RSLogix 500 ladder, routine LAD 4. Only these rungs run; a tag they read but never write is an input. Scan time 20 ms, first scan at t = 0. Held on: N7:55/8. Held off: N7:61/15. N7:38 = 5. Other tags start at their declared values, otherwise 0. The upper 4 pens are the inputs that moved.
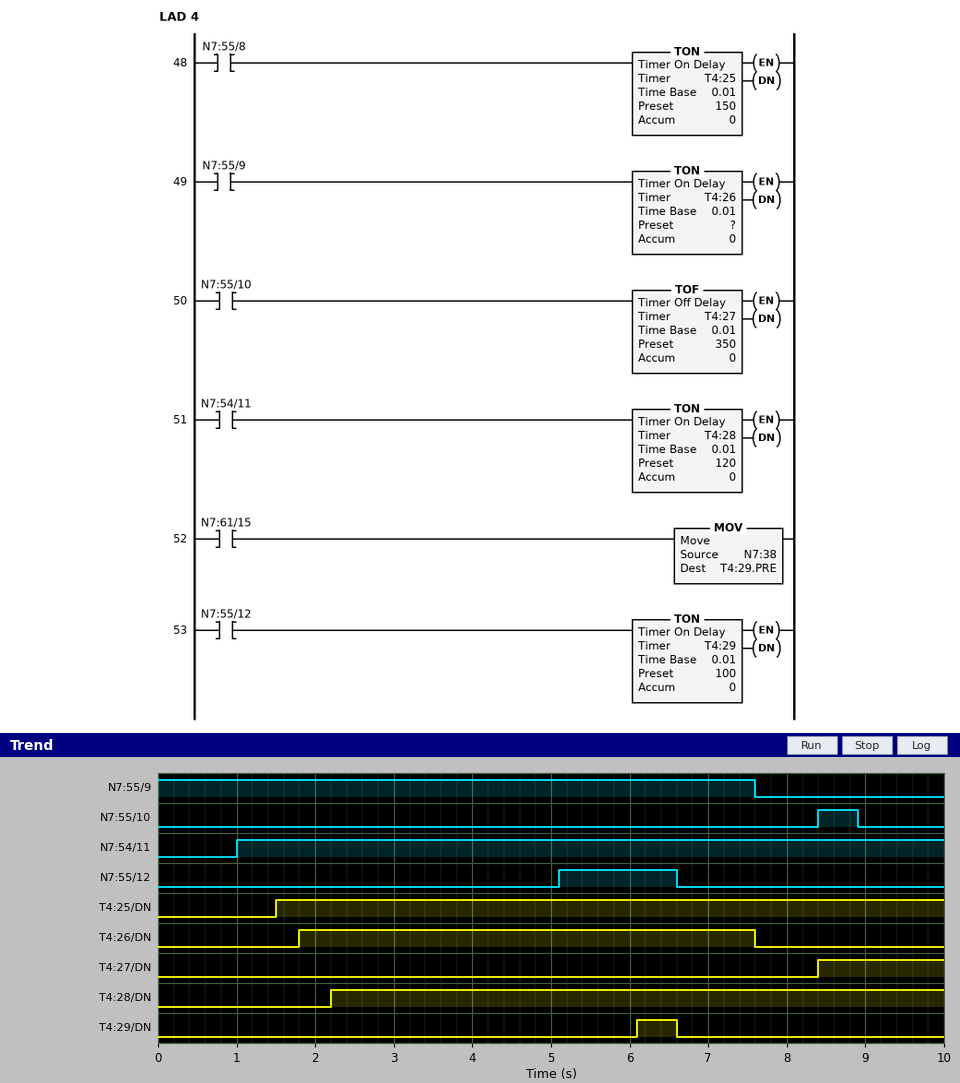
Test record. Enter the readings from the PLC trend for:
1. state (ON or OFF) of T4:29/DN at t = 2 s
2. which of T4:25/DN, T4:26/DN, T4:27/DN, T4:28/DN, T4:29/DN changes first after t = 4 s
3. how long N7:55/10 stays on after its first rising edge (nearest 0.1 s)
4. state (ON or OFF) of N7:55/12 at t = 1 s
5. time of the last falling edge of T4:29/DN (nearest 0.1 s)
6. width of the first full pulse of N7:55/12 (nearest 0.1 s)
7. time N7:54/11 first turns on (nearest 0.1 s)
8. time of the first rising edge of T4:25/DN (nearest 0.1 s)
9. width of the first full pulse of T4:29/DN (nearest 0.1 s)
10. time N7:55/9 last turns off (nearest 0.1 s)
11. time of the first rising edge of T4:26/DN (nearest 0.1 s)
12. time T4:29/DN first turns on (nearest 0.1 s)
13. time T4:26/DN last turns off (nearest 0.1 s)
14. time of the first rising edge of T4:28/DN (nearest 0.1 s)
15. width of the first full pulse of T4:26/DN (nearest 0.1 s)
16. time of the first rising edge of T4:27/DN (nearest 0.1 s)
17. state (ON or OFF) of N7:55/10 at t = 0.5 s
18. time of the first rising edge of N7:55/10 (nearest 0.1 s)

OFF
T4:29/DN
0.5 s
OFF
6.6 s
1.5 s
1.0 s
1.5 s
0.5 s
7.6 s
1.8 s
6.1 s
7.6 s
2.2 s
5.8 s
8.4 s
OFF
8.4 s
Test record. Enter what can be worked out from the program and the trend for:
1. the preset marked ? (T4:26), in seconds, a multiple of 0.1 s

1.8 s
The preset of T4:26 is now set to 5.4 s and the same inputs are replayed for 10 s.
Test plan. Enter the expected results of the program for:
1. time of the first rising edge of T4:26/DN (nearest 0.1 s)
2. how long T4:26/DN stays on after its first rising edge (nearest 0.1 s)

5.4 s
2.2 s
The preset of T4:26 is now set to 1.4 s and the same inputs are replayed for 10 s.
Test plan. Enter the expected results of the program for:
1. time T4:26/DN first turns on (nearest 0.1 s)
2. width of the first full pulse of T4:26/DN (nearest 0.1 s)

1.4 s
6.2 s
